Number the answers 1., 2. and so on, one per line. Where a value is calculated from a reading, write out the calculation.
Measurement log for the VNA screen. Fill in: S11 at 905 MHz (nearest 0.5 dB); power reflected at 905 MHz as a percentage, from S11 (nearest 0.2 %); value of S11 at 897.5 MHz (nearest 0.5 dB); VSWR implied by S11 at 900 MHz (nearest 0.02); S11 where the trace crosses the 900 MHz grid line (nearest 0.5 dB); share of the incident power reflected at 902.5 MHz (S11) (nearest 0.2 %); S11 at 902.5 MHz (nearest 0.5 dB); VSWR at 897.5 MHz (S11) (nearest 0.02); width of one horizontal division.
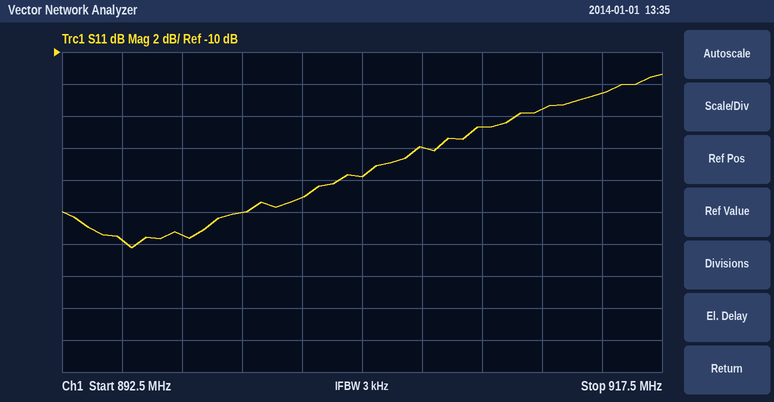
1. -18.0 dB
2. 10^(-18/10) ≈ 1.6 %
3. -21.5 dB
4. |Γ| = 10^(-20/20) = 0.1000; VSWR = (1 + 0.1000)/(1 − 0.1000) ≈ 1.22
5. -20.0 dB
6. 10^(-19/10) ≈ 1.26 %, so 1.2 % to the nearest 0.2 %
7. -19.0 dB
8. |Γ| = 10^(-21.5/20) = 0.0841; VSWR = (1 + 0.0841)/(1 − 0.0841) ≈ 1.18
9. 2.5 MHz
